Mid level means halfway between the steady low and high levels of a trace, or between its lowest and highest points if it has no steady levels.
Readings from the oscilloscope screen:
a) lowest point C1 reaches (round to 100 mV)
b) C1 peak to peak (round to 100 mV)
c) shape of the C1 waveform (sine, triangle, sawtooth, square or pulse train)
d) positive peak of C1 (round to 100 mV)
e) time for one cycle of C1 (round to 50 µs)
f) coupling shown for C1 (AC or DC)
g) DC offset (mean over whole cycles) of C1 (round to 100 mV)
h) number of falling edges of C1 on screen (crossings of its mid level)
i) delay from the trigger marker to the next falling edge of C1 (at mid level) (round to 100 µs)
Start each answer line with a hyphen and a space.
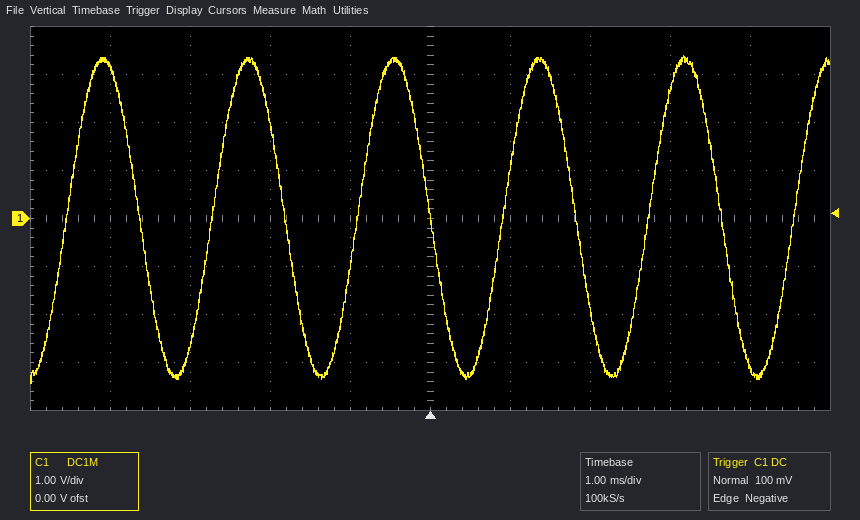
- -3.4 V
- 6.8 V
- sine
- 3.4 V
- 1.80 ms
- DC
- 0.0 V
- 5
- 1.8 ms
